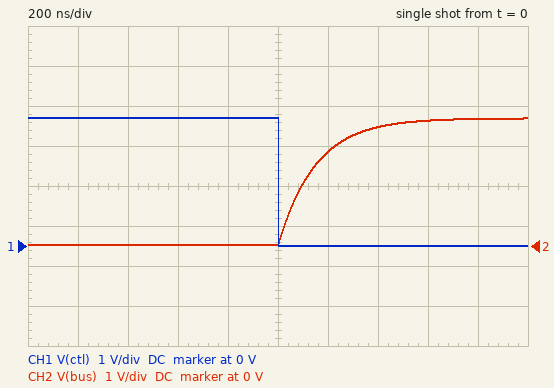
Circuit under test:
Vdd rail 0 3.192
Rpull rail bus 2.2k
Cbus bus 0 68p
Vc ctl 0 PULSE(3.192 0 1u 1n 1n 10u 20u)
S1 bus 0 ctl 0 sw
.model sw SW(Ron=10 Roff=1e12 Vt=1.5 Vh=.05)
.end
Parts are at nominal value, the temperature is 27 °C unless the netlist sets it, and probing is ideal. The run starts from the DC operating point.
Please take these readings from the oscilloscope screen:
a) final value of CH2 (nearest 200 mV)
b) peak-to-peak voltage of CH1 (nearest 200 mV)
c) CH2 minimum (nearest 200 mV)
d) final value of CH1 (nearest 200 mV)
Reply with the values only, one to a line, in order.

3.2 V
3.2 V
0 V
0 V
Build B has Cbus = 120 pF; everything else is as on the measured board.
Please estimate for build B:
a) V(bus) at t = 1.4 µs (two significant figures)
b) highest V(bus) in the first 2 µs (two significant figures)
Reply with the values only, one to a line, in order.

2.5 V
3.1 V
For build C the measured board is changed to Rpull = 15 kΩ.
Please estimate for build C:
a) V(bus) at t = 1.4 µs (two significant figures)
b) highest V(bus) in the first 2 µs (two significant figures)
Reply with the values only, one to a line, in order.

1.0 V
2.0 V
